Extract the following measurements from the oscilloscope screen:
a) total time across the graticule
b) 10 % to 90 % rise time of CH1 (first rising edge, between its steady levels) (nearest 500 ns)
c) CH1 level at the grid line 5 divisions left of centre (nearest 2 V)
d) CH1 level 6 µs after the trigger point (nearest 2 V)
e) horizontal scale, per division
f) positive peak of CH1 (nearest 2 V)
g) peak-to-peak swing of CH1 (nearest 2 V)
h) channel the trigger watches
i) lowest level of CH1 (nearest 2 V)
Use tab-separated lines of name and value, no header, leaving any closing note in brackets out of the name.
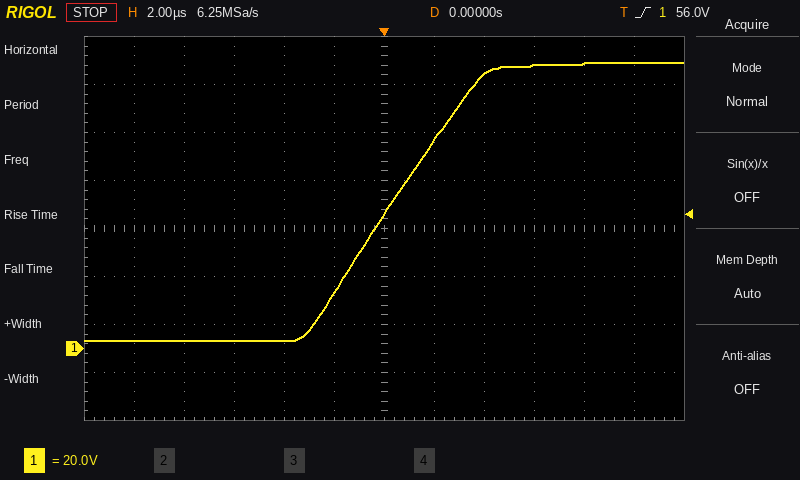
total time across the graticule	24 µs
10 % to 90 % rise time of CH1 (first rising edge, between its steady levels)	6.0 µs
CH1 level at the grid line 5 divisions left of centre	4 V
CH1 level 6 µs after the trigger point	118 V
horizontal scale, per division	2 µs
positive peak of CH1	120 V
peak-to-peak swing of CH1	116 V
channel the trigger watches	CH1
lowest level of CH1	4 V
